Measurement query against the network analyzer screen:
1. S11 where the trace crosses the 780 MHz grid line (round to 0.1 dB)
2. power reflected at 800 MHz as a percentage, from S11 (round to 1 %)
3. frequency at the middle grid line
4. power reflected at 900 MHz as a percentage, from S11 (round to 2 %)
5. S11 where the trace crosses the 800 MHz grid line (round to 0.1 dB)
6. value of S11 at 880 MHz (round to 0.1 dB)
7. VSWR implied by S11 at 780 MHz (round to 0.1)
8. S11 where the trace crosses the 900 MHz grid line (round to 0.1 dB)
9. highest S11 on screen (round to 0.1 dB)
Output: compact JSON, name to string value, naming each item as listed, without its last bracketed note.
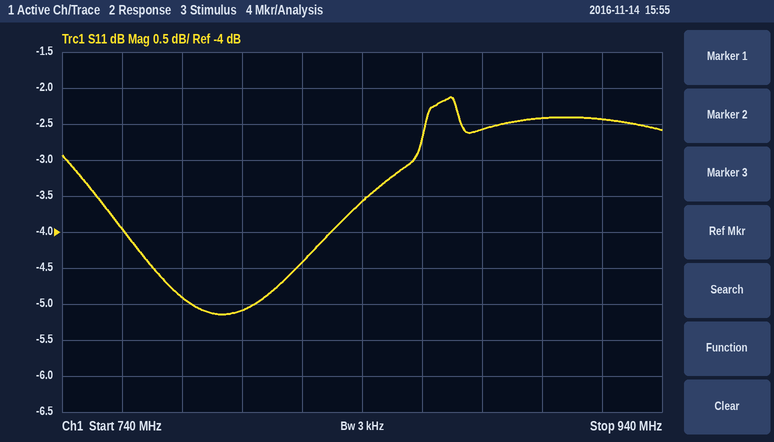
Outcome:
{"S11 where the trace crosses the 780 MHz grid line": "-4.9 dB", "power reflected at 800 MHz as a percentage, from S11": "31 %", "frequency at the middle grid line": "840 MHz", "power reflected at 900 MHz as a percentage, from S11": "58 %", "S11 where the trace crosses the 800 MHz grid line": "-5.1 dB", "value of S11 at 880 MHz": "-2.6 dB", "VSWR implied by S11 at 780 MHz": "3.6", "S11 where the trace crosses the 900 MHz grid line": "-2.4 dB", "highest S11 on screen": "-2.1 dB"}
